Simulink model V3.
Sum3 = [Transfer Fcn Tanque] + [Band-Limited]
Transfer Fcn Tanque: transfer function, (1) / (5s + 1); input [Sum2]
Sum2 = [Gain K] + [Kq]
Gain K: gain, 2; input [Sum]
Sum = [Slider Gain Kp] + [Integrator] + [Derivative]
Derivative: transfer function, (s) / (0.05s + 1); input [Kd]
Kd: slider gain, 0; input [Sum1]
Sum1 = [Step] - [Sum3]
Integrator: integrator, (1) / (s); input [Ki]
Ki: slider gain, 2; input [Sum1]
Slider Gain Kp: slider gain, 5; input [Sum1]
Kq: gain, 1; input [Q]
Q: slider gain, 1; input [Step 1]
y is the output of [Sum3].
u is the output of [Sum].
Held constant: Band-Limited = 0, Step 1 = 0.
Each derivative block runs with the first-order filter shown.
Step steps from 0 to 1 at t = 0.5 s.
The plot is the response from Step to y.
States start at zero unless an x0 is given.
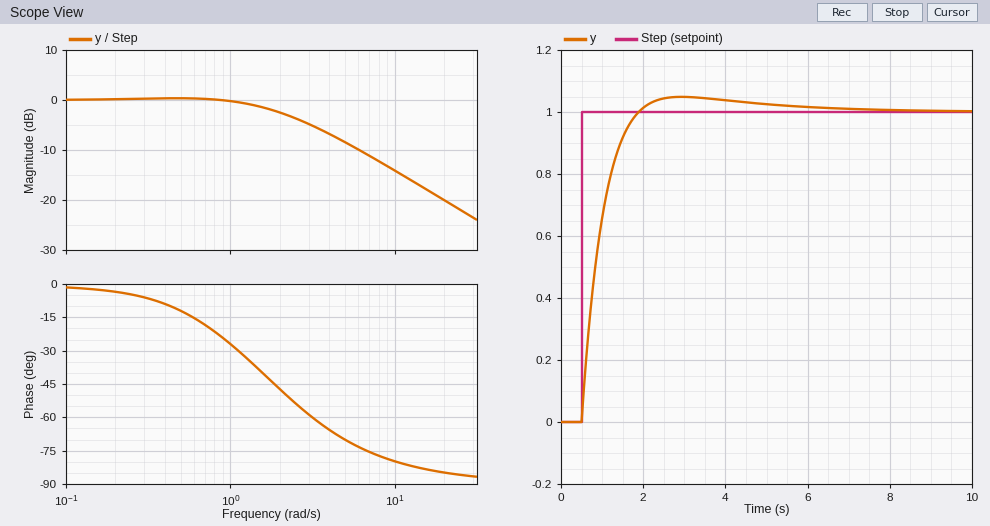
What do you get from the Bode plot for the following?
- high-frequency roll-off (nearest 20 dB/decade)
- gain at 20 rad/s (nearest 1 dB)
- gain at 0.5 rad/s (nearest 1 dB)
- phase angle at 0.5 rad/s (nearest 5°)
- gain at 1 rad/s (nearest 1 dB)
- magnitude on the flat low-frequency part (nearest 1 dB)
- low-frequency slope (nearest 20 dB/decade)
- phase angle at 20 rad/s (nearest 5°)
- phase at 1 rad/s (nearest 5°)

-20 dB/decade
-20 dB
0 dB
-10°
0 dB
0 dB
0 dB/decade
-85°
-25°
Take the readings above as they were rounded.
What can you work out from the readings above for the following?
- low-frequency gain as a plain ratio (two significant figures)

1.0
